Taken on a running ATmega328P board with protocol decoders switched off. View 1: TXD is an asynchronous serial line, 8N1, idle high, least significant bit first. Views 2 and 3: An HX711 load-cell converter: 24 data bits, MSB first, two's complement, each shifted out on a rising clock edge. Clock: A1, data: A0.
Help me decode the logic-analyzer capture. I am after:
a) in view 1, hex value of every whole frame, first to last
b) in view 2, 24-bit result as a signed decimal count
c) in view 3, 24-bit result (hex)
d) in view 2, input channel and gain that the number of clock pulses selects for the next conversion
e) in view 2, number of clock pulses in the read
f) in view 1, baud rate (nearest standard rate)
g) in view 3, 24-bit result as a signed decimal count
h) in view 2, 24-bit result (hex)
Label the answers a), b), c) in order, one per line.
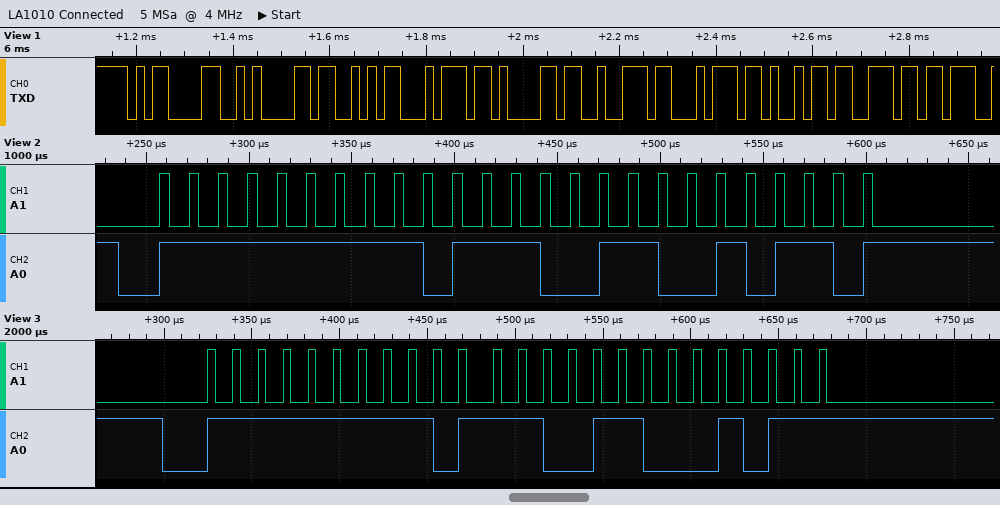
a) 0x0D 0x0A 0x53 0x74 0x61 0x72 0x74 0x69 0x6E
b) -18026
c) 0xFFB98B
d) channel A, gain 128
e) 25
f) 57600 baud
g) -18037
h) 0xFFB996
